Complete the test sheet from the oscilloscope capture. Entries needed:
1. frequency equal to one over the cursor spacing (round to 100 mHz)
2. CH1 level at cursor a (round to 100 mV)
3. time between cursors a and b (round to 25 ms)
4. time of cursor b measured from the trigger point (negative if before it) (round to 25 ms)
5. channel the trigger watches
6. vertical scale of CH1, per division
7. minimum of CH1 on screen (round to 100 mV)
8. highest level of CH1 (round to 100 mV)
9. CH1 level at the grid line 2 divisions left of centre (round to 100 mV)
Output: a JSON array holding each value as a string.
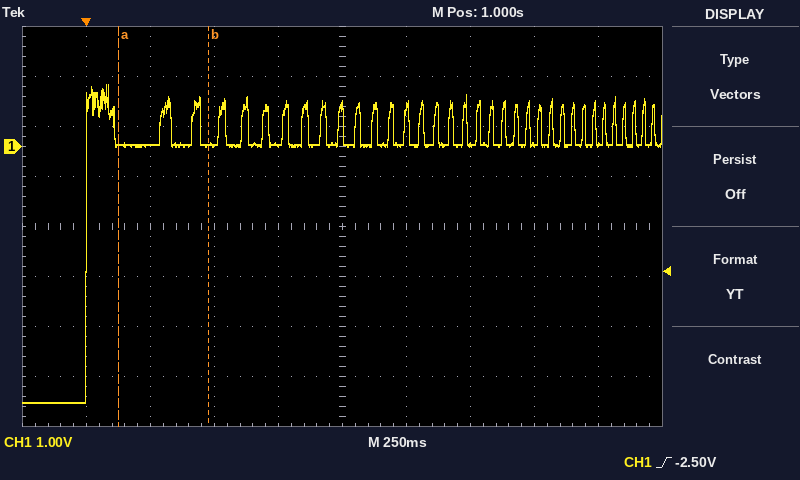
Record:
["2.9 Hz", "100 mV", "350 ms", "+475 ms", "CH1", "1 V", "-5.1 V", "1.2 V", "0.0 V"]
